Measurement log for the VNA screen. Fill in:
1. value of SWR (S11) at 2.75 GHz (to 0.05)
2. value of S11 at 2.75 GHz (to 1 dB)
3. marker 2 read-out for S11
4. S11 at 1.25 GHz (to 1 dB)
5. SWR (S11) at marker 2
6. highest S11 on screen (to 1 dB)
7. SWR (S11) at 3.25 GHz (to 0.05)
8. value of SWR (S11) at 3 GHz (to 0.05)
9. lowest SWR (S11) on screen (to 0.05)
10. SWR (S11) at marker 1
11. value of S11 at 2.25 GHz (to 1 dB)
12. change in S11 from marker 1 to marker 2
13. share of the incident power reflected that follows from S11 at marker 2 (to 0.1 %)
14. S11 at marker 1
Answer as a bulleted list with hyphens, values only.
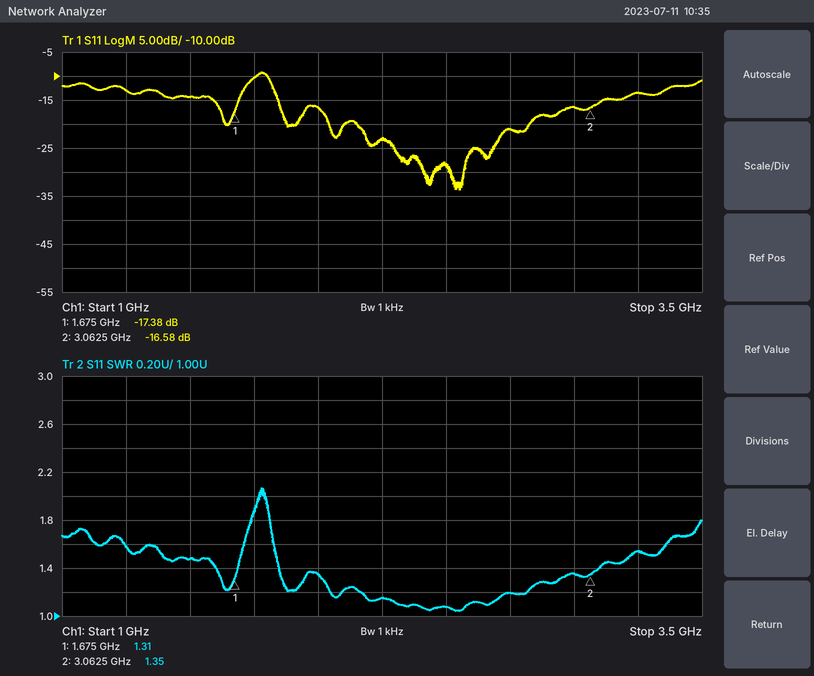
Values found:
- 1.20
- -21 dB
- -16.58 dB
- -13 dB
- 1.35
- -9 dB
- 1.55
- 1.35
- 1.05
- 1.31
- -23 dB
- 0.80 dB
- 2.2 %
- -17.38 dB
